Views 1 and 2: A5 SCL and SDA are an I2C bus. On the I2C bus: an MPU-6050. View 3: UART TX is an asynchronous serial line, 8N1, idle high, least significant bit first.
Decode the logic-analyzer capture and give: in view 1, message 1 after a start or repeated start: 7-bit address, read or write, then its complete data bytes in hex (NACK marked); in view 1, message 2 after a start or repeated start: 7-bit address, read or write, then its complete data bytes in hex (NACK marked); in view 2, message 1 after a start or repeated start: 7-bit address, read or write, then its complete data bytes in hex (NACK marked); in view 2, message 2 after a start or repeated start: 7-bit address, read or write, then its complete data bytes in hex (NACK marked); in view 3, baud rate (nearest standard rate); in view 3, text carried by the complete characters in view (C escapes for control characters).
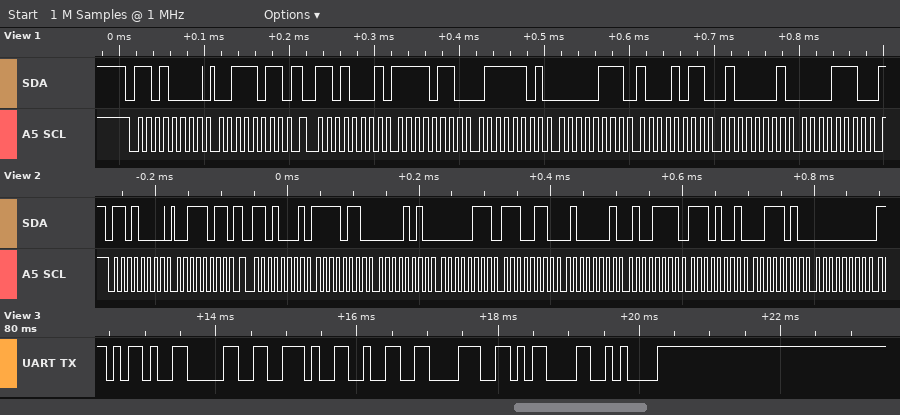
0x68 write: 3B
0x68 read: F6 7D 07 8B 41 0E
0x68 write: 3B
0x68 read: F6 0A 07 E6 41 4F E9 3A 00
9600 baud
"-0.28\r\n"
